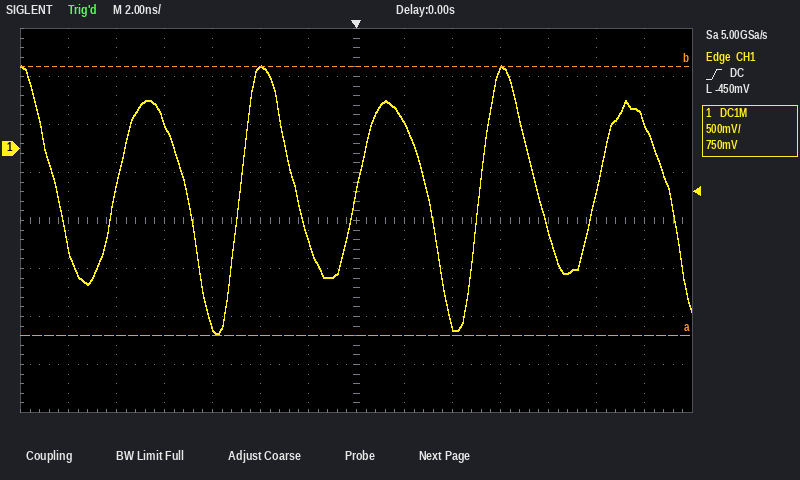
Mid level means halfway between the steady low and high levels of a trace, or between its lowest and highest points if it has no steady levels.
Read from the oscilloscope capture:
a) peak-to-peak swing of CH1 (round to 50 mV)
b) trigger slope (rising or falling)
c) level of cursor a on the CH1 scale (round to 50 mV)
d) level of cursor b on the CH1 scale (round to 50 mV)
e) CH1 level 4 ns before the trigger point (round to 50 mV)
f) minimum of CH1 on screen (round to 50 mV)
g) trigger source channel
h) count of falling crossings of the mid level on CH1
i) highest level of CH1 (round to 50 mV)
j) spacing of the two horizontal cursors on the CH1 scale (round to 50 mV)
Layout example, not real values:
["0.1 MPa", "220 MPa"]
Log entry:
["2.80 V", "rising", "-1.95 V", "850 mV", "850 mV", "-1.95 V", "CH1", "6", "850 mV", "2.80 V"]
